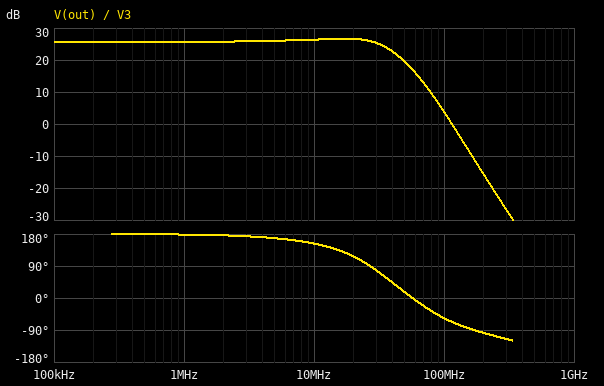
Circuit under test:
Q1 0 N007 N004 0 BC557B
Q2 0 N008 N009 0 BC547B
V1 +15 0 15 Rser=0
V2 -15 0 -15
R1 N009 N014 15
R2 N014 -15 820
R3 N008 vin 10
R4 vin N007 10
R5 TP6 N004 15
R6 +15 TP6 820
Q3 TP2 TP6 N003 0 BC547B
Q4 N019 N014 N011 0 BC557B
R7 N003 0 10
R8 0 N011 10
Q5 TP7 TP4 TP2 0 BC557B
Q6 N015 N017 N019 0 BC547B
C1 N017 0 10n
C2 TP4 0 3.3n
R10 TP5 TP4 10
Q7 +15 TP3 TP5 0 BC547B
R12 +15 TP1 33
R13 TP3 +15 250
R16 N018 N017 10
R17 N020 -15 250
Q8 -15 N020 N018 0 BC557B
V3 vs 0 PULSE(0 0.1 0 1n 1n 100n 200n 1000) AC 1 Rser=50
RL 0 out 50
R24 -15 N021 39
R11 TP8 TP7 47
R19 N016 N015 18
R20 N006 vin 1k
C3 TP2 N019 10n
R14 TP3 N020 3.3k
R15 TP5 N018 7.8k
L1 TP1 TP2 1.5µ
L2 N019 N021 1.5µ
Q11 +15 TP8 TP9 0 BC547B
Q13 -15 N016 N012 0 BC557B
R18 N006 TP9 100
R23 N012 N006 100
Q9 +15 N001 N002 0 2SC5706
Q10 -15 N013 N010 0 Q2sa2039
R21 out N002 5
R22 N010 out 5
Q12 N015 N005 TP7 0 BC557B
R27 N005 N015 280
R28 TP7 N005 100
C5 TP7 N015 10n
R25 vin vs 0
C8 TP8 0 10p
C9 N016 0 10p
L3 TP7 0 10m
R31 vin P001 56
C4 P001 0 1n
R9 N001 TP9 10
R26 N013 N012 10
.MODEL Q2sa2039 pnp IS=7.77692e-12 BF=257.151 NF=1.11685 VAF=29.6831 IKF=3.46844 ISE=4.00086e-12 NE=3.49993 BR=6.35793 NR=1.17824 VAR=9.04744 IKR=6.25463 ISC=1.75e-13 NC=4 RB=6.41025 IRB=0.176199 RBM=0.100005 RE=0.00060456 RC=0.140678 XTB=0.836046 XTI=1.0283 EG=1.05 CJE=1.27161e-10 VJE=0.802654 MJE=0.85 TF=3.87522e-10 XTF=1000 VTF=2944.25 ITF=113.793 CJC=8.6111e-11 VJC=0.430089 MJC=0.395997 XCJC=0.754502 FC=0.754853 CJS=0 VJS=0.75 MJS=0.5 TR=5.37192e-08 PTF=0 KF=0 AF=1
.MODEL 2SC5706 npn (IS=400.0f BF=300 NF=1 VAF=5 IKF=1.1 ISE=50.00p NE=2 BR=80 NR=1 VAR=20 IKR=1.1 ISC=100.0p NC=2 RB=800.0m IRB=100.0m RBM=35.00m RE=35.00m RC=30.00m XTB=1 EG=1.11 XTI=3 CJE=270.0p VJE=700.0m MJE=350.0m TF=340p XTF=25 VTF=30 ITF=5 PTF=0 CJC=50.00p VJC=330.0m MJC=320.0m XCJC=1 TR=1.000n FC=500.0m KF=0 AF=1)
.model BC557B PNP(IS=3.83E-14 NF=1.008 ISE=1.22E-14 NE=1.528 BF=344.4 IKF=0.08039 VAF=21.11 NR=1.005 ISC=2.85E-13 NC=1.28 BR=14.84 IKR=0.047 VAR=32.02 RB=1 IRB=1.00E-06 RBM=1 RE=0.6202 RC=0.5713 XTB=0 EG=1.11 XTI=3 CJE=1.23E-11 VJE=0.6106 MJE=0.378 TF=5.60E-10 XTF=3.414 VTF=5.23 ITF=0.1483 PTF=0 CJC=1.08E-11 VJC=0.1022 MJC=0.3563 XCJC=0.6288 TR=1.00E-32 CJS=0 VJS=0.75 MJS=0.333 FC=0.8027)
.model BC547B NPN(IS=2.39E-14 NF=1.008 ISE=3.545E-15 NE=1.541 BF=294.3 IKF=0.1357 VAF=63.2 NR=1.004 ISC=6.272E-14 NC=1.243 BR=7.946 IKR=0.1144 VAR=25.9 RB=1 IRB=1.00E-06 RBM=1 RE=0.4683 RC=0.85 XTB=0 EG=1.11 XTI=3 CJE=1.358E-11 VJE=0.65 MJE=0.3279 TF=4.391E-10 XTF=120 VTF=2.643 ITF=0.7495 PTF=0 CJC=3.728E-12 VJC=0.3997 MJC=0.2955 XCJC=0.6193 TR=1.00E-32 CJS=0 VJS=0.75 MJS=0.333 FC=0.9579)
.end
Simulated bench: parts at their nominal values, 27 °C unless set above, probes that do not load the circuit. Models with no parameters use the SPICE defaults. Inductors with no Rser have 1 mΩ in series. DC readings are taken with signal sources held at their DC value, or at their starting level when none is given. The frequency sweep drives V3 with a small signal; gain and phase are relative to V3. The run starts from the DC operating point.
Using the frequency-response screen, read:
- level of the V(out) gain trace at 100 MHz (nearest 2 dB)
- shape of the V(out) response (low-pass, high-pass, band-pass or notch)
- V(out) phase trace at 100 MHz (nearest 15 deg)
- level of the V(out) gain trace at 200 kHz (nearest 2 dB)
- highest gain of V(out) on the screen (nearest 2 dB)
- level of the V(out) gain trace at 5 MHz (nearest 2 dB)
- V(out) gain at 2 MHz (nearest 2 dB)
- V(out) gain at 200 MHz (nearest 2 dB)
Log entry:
4 dB
low-pass
-60 deg
26 dB
26 dB
26 dB
26 dB
-16 dB
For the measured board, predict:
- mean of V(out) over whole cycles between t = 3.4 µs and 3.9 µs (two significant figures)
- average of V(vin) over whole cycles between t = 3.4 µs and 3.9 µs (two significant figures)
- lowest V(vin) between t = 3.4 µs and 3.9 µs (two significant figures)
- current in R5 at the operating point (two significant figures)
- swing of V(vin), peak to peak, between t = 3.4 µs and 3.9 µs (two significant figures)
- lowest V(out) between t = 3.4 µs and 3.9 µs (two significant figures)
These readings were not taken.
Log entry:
-2.1 V
-58 mV
-110 mV
17 mA
100 mV
-3.3 V
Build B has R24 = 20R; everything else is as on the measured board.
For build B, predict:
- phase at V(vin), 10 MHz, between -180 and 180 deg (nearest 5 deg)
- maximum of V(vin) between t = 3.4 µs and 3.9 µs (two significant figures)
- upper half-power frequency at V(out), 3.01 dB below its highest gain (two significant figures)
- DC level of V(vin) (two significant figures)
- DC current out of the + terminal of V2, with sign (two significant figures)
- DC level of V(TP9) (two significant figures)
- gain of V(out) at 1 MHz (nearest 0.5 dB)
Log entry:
75 deg
-14 mV
41 MHz
-69 mV
-180 mA
-690 mV
26.0 dB
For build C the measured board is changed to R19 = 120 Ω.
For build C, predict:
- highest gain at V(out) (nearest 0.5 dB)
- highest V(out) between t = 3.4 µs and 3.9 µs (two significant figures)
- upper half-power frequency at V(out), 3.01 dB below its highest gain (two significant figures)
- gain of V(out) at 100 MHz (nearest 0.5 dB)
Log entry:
27.5 dB
-700 mV
33 MHz
1.5 dB
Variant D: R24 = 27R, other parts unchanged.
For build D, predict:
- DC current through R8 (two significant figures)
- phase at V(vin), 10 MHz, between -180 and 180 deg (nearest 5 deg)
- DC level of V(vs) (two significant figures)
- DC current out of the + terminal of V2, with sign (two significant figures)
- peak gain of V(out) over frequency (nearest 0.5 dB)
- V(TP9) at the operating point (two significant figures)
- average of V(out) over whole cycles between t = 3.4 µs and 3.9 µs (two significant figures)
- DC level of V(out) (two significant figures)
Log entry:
31 mA
75 deg
-65 mV
-140 mA
27.0 dB
-690 mV
-2.3 V
-1.3 V
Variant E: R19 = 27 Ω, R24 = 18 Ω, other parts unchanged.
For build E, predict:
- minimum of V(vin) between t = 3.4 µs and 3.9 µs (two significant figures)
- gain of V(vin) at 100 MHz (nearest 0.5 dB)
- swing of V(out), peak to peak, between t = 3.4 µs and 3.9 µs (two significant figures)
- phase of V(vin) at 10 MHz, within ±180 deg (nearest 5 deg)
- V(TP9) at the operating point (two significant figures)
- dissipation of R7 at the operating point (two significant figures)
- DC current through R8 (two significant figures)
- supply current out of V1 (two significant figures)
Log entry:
-120 mV
-7.5 dB
2.6 V
75 deg
-690 mV
3.3 mW
32 mA
120 mA
